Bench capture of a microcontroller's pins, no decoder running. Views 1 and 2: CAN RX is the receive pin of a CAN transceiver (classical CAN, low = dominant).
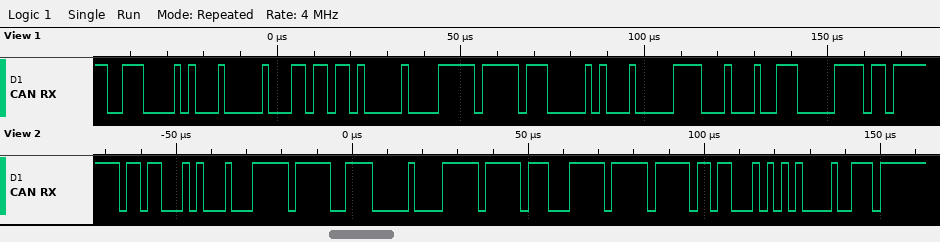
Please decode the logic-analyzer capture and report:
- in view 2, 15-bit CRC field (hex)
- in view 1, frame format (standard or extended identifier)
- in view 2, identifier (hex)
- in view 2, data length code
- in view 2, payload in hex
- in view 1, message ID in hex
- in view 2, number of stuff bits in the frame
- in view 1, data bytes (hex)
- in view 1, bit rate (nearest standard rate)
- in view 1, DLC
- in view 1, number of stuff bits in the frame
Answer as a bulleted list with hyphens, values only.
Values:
- 0x2A13
- standard
- 0x6C5
- 8
- FF DE 00 FF F8 FF FF B1
- 0x385
- 8
- 06 DA 00 FF F8 11 07 11
- 500 kbit/s
- 8
- 7
